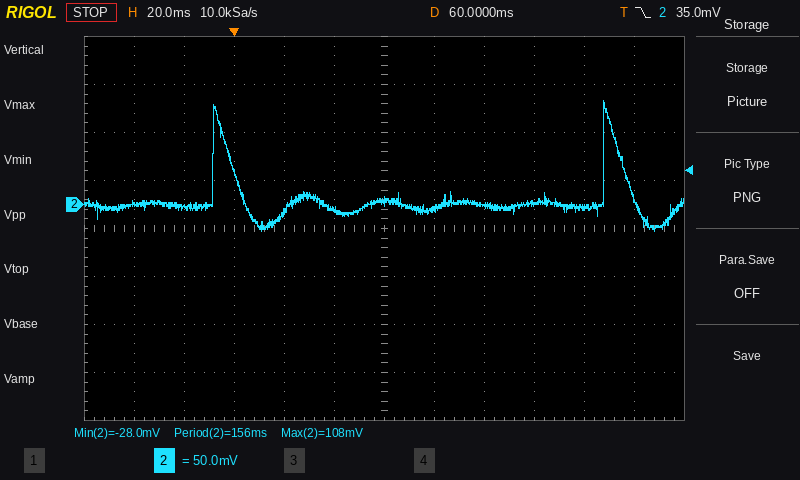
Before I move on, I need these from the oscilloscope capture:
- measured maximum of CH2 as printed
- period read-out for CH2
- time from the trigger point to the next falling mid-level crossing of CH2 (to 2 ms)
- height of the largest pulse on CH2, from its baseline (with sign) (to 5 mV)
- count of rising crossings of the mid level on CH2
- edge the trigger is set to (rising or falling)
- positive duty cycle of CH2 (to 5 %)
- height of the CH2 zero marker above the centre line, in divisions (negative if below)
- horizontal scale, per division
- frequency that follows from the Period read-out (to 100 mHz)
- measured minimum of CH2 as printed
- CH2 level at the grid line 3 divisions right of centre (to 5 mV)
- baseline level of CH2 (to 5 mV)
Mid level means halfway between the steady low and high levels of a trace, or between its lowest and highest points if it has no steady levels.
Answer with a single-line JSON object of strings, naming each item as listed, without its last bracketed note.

{"measured maximum of CH2 as printed": "108 mV", "period read-out for CH2": "156 ms", "time from the trigger point to the next falling mid-level crossing of CH2": "156 ms", "height of the largest pulse on CH2, from its baseline (with sign)": "+110 mV", "count of rising crossings of the mid level on CH2": "2", "edge the trigger is set to": "falling", "positive duty cycle of CH2": "5 %", "height of the CH2 zero marker above the centre line, in divisions": "+0.5 div", "horizontal scale, per division": "20 ms", "frequency that follows from the Period read-out": "6.4 Hz", "measured minimum of CH2 as printed": "-28.0 mV", "CH2 level at the grid line 3 divisions right of centre": "0 mV", "baseline level of CH2": "0 mV"}
